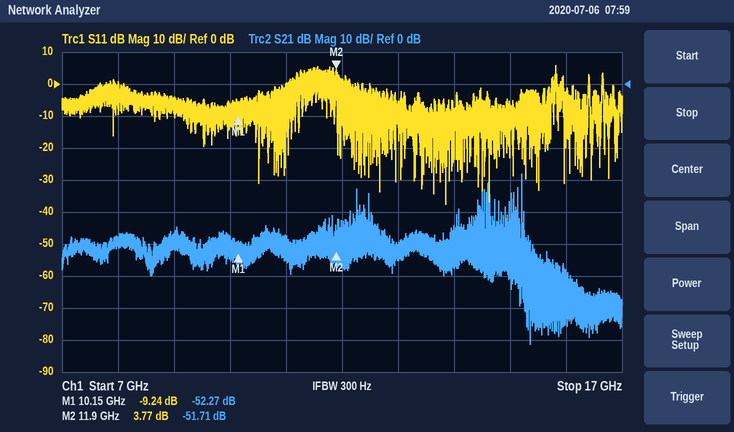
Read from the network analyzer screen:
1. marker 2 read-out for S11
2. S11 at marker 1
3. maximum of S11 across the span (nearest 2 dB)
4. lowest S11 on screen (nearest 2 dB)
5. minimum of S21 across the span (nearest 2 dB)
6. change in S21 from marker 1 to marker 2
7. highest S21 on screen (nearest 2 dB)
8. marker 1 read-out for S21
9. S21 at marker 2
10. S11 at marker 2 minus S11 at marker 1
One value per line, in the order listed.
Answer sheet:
3.77 dB
-9.24 dB
6 dB
-38 dB
-82 dB
0.56 dB
-28 dB
-52.27 dB
-51.71 dB
13.01 dB
